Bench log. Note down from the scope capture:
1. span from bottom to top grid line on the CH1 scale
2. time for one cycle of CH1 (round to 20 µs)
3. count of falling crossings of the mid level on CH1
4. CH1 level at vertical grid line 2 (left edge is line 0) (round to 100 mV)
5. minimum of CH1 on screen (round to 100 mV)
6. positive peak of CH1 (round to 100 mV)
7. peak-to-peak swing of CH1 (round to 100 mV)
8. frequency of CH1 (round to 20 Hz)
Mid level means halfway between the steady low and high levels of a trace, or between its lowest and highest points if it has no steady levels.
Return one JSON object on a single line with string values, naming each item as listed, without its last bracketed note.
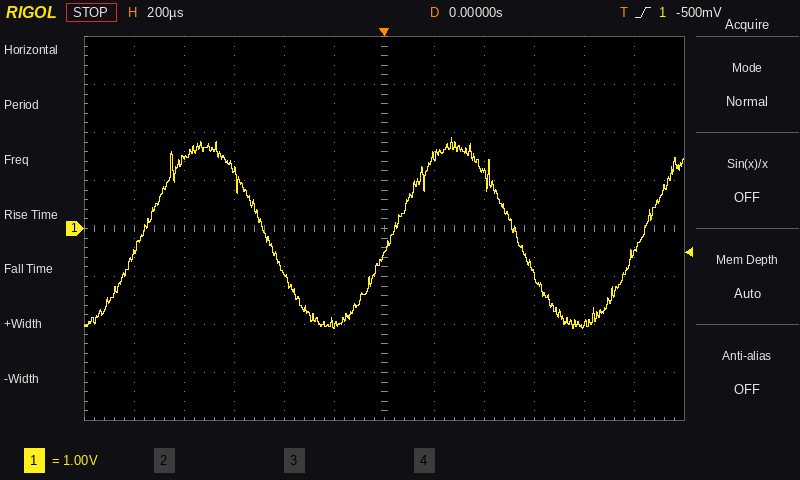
{"span from bottom to top grid line on the CH1 scale": "8 V", "time for one cycle of CH1": "1.00 ms", "count of falling crossings of the mid level on CH1": "2", "CH1 level at vertical grid line 2 (left edge is line 0)": "1.4 V", "minimum of CH1 on screen": "-2.1 V", "positive peak of CH1": "1.9 V", "peak-to-peak swing of CH1": "4.0 V", "frequency of CH1": "1.00 kHz"}
